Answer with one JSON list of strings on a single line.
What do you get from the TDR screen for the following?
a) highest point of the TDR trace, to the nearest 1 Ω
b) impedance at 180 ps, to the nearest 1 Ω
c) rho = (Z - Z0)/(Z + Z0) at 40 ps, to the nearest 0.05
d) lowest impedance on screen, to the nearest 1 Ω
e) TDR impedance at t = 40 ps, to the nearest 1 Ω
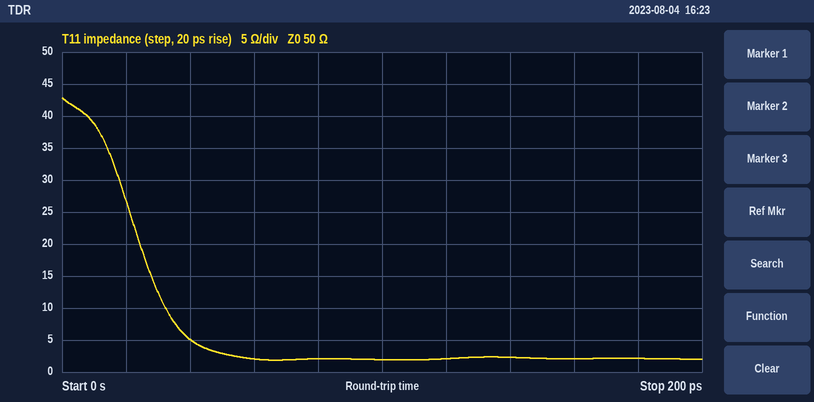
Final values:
["43 Ω", "2 Ω", "-0.80", "2 Ω", "5 Ω"]
